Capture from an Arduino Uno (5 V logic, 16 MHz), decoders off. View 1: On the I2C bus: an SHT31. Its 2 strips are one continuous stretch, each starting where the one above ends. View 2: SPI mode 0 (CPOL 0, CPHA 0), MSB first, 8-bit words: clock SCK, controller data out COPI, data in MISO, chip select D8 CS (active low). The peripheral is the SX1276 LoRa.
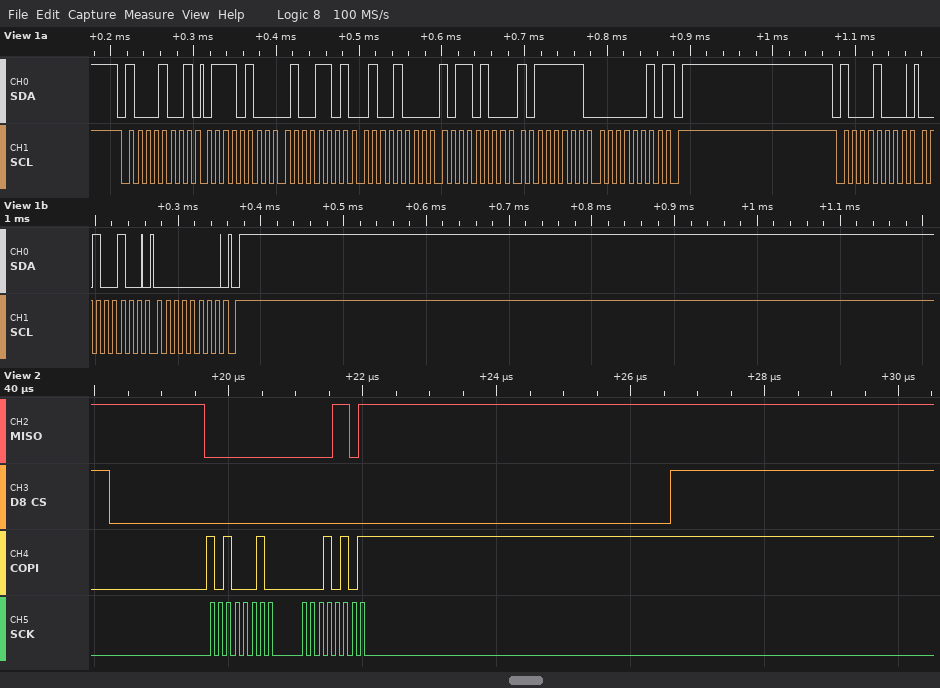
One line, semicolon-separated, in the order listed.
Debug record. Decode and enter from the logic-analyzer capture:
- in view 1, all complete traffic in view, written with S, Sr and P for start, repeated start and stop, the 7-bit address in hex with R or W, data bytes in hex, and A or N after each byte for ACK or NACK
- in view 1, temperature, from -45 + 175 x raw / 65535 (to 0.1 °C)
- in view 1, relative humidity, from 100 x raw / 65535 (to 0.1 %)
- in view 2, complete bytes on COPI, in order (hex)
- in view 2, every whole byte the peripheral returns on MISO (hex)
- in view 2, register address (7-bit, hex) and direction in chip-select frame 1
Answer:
S 44R A 74 A 4D A 48 A B4 A BF A 02 N P S 44W A 24 A 00 A P; 34.5 °C; 70.6 %; A2 15; 00 0D; 0x22 write
